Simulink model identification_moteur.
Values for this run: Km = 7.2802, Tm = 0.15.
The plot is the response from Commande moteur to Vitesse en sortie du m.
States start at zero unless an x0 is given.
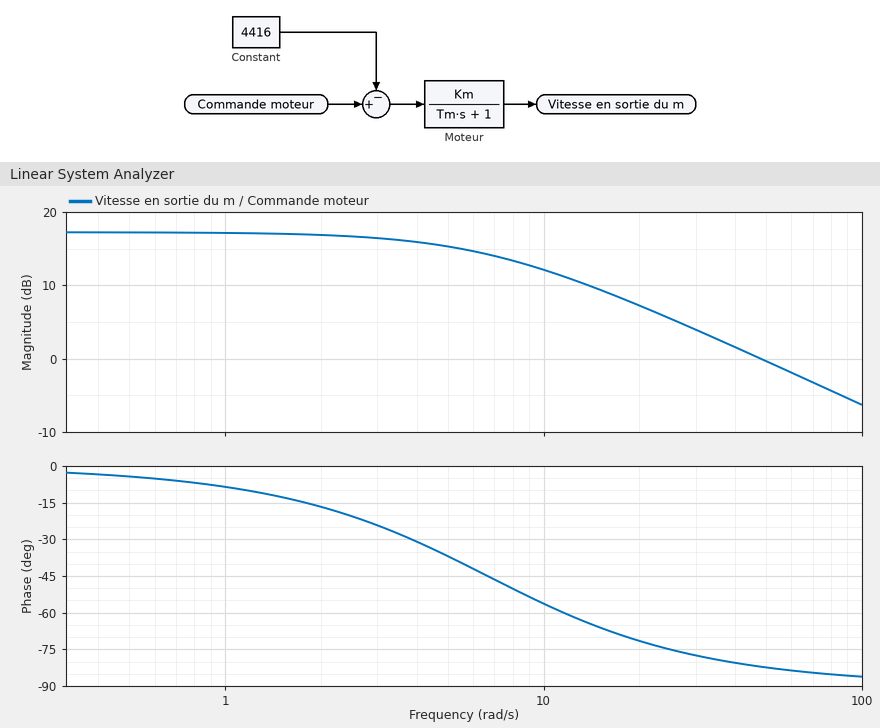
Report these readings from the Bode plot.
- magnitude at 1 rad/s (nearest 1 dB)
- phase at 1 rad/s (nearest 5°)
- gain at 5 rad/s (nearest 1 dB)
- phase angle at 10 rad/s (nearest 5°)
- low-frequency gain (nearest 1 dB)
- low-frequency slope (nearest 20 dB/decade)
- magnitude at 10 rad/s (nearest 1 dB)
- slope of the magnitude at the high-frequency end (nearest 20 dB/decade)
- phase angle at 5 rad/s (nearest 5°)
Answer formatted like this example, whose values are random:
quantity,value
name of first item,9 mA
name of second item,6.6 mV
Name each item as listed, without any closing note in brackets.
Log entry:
quantity,value
magnitude at 1 rad/s,17 dB
phase at 1 rad/s,-10°
gain at 5 rad/s,15 dB
phase angle at 10 rad/s,-55°
low-frequency gain,17 dB
low-frequency slope,0 dB/decade
magnitude at 10 rad/s,12 dB
slope of the magnitude at the high-frequency end,-20 dB/decade
phase angle at 5 rad/s,-35°
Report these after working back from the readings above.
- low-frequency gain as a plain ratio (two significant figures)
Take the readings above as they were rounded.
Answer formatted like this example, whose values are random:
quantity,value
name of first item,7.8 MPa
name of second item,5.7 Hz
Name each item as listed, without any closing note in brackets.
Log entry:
quantity,value
low-frequency gain as a plain ratio,7.1
